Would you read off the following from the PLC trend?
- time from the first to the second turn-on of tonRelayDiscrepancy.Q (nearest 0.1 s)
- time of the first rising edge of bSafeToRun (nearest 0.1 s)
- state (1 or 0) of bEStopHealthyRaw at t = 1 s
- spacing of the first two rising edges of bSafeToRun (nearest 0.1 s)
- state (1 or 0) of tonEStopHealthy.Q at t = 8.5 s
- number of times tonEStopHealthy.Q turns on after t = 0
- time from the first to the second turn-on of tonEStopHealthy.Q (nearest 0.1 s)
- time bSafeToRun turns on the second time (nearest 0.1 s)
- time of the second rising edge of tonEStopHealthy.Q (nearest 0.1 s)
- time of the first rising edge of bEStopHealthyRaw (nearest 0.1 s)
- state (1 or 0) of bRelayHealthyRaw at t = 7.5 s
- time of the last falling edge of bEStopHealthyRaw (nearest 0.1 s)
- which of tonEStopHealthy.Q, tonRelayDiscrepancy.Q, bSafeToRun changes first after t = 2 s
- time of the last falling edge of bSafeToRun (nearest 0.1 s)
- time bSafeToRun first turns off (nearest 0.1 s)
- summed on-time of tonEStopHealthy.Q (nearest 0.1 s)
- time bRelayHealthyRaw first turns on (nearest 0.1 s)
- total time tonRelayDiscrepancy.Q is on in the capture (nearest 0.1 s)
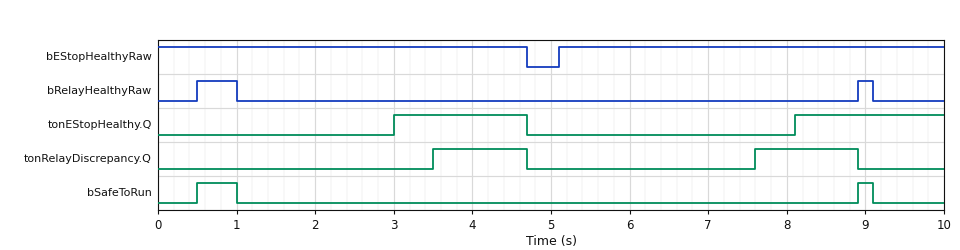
4.1 s
0.5 s
1
8.4 s
1
2
5.1 s
8.9 s
8.1 s
5.1 s
0
4.7 s
tonEStopHealthy.Q
9.1 s
1.0 s
3.6 s
0.5 s
2.5 s
